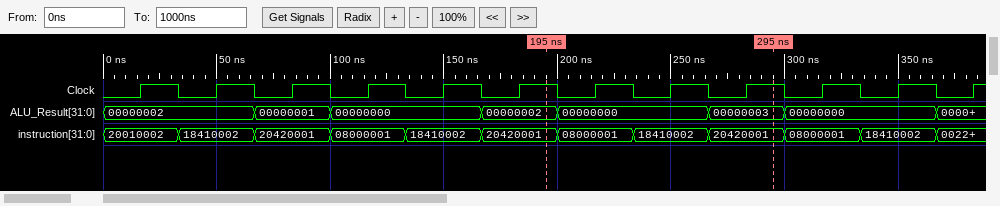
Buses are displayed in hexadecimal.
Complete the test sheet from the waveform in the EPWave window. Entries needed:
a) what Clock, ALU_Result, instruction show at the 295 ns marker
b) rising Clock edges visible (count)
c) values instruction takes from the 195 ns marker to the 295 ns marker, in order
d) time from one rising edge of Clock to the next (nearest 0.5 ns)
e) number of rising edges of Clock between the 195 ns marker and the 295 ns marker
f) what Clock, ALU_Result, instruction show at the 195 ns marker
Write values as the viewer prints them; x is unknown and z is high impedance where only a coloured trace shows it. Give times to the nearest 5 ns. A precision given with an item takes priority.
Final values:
Clock=1, ALU_Result=00000003, instruction=20420001
12
20420001, 08000001, 18410002, 20420001
33.5 ns
3
Clock=1, ALU_Result=00000002, instruction=20420001
